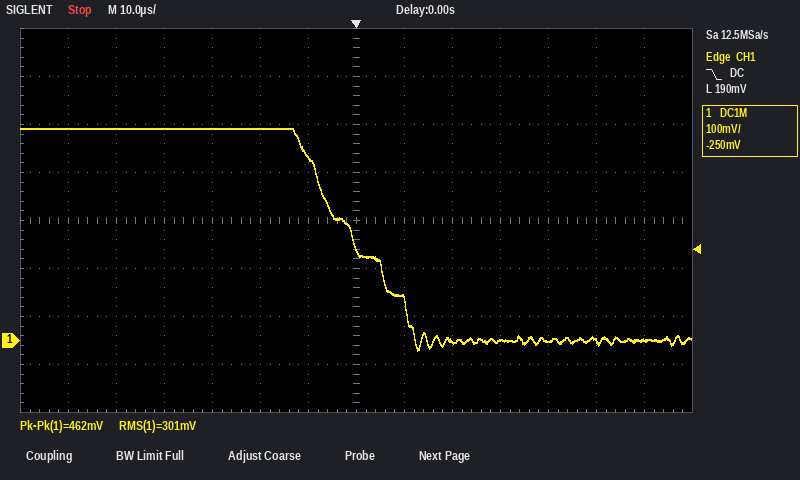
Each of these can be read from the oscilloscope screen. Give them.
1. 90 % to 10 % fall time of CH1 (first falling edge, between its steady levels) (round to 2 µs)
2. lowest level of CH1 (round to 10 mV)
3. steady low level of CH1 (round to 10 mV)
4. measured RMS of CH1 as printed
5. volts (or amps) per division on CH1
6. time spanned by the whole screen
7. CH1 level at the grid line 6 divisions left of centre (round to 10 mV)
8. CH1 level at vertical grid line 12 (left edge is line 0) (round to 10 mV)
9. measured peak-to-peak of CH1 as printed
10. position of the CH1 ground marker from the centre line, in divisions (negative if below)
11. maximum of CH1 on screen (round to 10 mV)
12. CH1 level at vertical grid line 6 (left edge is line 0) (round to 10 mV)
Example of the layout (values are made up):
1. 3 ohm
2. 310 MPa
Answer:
1. 22 µs
2. -20 mV
3. 0 mV
4. 301 mV
5. 100 mV
6. 140 µs
7. 440 mV
8. 0 mV
9. 462 mV
10. -2.5 div
11. 440 mV
12. 380 mV
